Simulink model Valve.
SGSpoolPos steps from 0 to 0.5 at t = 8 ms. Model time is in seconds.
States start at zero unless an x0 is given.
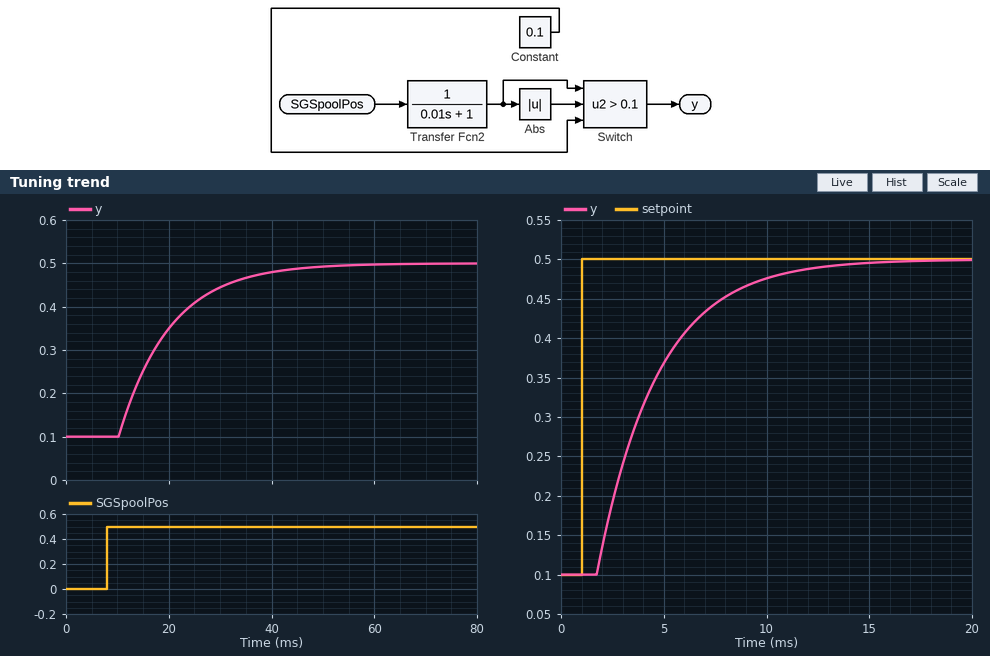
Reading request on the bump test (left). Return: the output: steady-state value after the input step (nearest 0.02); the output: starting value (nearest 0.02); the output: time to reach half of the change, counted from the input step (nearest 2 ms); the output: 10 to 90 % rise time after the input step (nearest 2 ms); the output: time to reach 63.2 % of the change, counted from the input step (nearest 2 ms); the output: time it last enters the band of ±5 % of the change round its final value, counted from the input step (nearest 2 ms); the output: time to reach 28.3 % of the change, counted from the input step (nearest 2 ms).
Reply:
0.50
0.10
10 ms
22 ms
12 ms
32 ms
6 ms
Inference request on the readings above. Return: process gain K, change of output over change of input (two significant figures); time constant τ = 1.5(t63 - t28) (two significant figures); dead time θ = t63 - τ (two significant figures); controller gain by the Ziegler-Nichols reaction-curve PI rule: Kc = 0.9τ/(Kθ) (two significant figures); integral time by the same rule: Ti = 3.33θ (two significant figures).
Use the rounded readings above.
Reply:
0.80
9.0 ms
3.0 ms
3.4
10.0 ms
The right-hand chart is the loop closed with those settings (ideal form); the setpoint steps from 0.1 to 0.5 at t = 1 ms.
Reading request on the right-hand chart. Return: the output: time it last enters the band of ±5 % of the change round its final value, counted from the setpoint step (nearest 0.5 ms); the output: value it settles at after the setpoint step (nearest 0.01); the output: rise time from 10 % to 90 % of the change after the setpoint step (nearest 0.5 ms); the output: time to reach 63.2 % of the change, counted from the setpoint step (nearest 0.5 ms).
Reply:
9.5 ms
0.50
6.5 ms
3.5 ms
